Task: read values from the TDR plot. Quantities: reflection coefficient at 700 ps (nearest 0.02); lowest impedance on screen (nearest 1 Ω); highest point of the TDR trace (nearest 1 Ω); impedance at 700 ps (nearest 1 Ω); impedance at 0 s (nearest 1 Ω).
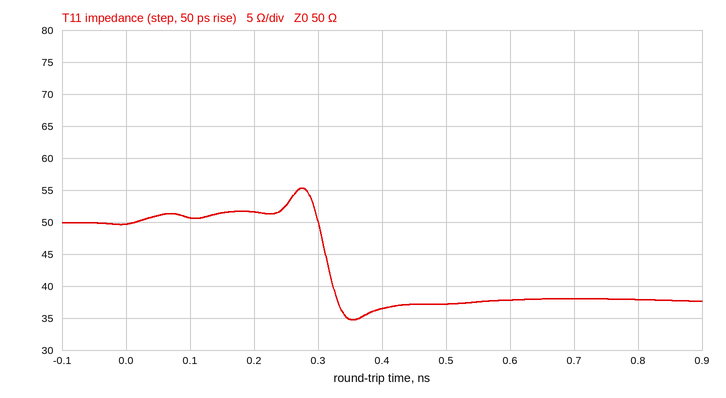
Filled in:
-0.14
35 Ω
55 Ω
38 Ω
50 Ω
